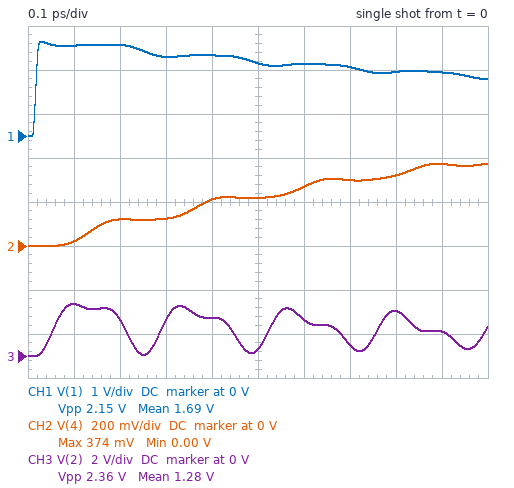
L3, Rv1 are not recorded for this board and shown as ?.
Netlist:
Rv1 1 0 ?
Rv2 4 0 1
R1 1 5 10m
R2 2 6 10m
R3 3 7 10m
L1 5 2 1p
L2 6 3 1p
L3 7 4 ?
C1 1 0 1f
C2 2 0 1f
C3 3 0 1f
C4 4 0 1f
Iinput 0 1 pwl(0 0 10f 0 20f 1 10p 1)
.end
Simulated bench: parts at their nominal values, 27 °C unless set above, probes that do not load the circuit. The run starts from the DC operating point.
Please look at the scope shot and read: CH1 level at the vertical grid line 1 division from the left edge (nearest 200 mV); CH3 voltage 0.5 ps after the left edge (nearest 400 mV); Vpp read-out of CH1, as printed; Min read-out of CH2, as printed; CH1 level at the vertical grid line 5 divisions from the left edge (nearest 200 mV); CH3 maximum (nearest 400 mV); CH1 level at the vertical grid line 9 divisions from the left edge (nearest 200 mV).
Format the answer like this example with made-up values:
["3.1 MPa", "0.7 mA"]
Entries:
["2.0 V", "400 mV", "2.15 V", "0.00 V", "1.6 V", "2.4 V", "1.4 V"]
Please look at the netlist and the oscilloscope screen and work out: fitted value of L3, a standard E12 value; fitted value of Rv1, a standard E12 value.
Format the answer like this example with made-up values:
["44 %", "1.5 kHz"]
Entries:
["1.8 pH", "2.2 Ω"]
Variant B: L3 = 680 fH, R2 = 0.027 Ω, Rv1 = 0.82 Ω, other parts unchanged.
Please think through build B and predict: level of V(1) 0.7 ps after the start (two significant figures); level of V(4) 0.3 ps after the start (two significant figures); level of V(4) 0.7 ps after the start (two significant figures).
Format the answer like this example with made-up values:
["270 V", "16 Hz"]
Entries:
["690 mV", "82 mV", "180 mV"]
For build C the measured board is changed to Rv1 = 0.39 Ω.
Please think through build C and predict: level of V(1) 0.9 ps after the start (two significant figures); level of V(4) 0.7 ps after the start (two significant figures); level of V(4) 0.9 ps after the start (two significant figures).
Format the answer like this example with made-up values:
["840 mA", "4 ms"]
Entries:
["360 mV", "62 mV", "81 mV"]
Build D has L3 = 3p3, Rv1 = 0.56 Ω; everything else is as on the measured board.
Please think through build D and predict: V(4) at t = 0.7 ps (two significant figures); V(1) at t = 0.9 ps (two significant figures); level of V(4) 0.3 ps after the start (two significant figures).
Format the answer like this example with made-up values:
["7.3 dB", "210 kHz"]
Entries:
["69 mV", "510 mV", "26 mV"]
